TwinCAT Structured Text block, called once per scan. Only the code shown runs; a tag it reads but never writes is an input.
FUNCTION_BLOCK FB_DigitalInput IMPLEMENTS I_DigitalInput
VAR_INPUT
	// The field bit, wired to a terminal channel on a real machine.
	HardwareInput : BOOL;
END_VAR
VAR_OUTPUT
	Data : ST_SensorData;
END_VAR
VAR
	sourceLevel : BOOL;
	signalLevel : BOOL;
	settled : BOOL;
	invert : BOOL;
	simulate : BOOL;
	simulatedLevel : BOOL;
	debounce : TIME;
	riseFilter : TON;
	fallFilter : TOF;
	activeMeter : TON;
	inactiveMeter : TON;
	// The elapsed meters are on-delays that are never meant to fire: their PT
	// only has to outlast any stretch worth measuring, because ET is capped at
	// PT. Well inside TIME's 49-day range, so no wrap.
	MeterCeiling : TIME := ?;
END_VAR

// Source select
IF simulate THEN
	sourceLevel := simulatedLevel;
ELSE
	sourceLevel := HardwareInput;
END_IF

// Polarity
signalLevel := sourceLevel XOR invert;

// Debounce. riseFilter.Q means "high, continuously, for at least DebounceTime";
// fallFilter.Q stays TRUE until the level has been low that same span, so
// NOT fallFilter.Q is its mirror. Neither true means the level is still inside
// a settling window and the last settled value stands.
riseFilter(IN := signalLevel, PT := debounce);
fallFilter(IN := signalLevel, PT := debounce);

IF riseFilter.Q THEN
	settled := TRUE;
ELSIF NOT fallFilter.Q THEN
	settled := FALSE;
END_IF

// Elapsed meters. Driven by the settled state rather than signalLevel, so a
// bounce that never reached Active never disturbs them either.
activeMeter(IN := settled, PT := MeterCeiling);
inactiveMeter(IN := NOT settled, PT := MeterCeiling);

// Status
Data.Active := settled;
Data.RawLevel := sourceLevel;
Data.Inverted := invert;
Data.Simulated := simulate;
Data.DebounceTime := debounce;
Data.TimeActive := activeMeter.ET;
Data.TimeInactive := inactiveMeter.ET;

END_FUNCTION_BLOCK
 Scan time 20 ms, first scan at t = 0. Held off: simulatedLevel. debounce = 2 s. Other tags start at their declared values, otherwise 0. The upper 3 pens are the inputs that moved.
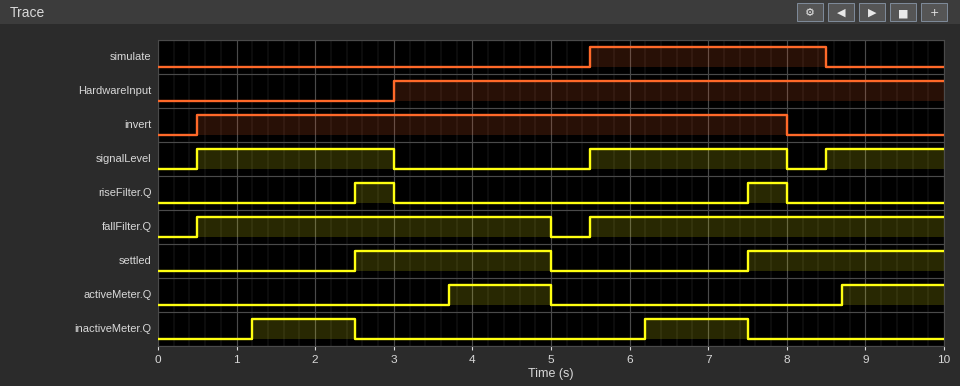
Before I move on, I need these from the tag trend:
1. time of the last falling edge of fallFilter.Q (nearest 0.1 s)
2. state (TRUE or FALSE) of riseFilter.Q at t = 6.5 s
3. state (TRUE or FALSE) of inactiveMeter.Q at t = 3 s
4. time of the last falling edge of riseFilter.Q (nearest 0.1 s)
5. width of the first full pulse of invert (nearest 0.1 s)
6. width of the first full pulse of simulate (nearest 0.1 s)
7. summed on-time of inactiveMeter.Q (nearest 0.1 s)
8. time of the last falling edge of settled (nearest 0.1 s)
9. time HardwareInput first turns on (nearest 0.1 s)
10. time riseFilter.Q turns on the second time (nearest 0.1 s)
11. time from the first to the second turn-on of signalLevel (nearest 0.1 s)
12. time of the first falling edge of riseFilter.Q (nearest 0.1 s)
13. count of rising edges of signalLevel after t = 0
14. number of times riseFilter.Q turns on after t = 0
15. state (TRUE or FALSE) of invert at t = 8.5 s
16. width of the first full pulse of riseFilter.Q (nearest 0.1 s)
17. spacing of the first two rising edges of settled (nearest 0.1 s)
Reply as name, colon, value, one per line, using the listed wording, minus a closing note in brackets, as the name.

time of the last falling edge of fallFilter.Q: 5.0 s
state (TRUE or FALSE) of riseFilter.Q at t = 6.5 s: FALSE
state (TRUE or FALSE) of inactiveMeter.Q at t = 3 s: FALSE
time of the last falling edge of riseFilter.Q: 8.0 s
width of the first full pulse of invert: 7.5 s
width of the first full pulse of simulate: 3.0 s
summed on-time of inactiveMeter.Q: 2.6 s
time of the last falling edge of settled: 5.0 s
time HardwareInput first turns on: 3.0 s
time riseFilter.Q turns on the second time: 7.5 s
time from the first to the second turn-on of signalLevel: 5.0 s
time of the first falling edge of riseFilter.Q: 3.0 s
count of rising edges of signalLevel after t = 0: 3
number of times riseFilter.Q turns on after t = 0: 2
state (TRUE or FALSE) of invert at t = 8.5 s: FALSE
width of the first full pulse of riseFilter.Q: 0.5 s
spacing of the first two rising edges of settled: 5.0 s
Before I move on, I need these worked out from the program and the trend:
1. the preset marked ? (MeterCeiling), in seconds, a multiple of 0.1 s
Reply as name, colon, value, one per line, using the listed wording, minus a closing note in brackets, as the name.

the preset marked ? (MeterCeiling), in seconds, a multiple of 0.1 s: 1.2 s
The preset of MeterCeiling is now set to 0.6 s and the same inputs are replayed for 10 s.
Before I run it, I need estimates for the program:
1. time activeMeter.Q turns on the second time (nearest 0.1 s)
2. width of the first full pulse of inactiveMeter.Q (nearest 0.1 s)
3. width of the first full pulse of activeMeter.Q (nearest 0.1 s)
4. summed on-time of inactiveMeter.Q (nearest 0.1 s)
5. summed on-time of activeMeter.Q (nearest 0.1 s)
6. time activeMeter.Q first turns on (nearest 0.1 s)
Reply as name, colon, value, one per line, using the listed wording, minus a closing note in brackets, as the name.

time activeMeter.Q turns on the second time: 8.1 s
width of the first full pulse of inactiveMeter.Q: 1.9 s
width of the first full pulse of activeMeter.Q: 1.9 s
summed on-time of inactiveMeter.Q: 3.8 s
summed on-time of activeMeter.Q: 3.8 s
time activeMeter.Q first turns on: 3.1 s
